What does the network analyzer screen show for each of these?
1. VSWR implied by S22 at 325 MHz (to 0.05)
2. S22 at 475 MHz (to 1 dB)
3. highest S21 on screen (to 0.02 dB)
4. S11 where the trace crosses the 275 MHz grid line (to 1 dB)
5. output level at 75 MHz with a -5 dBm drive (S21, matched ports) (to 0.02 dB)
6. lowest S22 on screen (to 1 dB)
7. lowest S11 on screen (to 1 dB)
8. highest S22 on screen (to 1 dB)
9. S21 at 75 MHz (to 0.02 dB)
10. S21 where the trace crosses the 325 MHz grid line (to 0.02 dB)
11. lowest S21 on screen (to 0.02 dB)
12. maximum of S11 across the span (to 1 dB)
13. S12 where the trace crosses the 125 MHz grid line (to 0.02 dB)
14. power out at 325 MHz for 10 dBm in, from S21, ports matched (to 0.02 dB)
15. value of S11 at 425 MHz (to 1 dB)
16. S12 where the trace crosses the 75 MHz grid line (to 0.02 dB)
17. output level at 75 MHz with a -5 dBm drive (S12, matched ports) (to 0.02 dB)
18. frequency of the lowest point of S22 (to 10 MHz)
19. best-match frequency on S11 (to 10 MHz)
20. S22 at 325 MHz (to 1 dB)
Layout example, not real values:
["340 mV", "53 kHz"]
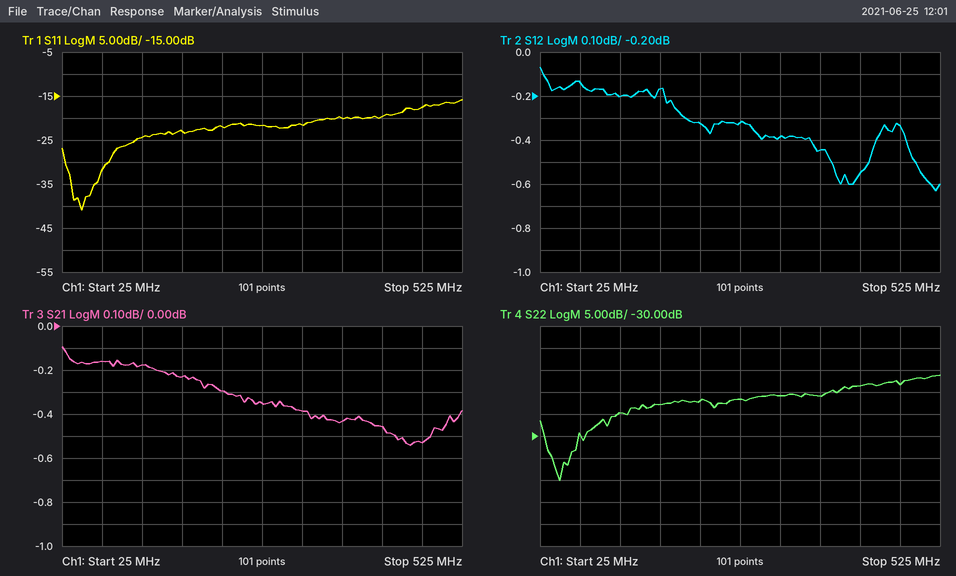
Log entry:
["1.20", "-18 dB", "-0.10 dB", "-22 dB", "-5.16 dBm", "-40 dB", "-41 dB", "-16 dB", "-0.16 dB", "-0.38 dB", "-0.54 dB", "-16 dB", "-0.20 dB", "9.62 dBm", "-20 dB", "-0.14 dB", "-5.14 dBm", "50 MHz", "50 MHz", "-21 dB"]
